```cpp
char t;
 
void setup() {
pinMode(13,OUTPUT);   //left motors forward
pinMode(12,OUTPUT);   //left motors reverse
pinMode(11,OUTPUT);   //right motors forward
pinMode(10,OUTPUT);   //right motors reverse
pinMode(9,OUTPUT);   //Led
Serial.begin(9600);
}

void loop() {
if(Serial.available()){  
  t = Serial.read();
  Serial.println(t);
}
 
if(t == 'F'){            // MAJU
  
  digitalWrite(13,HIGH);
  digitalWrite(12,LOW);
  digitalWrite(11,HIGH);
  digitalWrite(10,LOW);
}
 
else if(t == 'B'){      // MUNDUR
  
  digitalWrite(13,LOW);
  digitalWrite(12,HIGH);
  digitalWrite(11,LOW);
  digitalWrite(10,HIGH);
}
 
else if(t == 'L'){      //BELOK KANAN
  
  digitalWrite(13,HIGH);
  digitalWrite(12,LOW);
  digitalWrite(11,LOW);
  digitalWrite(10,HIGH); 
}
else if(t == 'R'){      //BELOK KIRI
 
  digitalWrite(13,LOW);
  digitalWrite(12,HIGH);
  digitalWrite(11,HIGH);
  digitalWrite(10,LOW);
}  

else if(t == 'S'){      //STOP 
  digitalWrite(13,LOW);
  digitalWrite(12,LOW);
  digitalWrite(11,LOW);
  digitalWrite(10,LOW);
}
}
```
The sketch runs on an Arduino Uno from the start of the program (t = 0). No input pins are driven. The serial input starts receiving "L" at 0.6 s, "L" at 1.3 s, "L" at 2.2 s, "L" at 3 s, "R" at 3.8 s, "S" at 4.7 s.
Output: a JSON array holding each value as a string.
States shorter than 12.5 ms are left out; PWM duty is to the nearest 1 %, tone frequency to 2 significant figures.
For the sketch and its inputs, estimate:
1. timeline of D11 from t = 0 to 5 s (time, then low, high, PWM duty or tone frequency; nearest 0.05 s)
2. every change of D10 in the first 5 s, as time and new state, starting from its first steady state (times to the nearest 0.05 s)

["0 s low; 3.8 s high; 4.7 s low", "0 s low; 0.6 s high; 3.8 s low"]
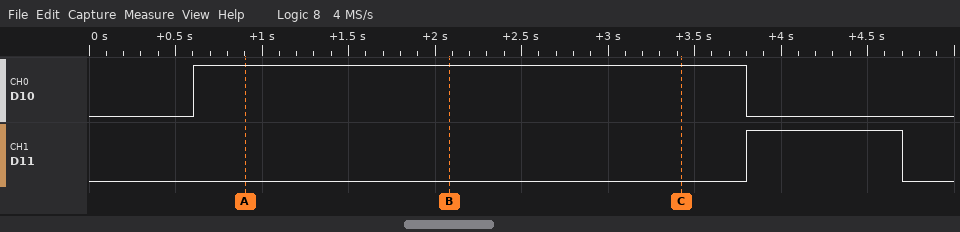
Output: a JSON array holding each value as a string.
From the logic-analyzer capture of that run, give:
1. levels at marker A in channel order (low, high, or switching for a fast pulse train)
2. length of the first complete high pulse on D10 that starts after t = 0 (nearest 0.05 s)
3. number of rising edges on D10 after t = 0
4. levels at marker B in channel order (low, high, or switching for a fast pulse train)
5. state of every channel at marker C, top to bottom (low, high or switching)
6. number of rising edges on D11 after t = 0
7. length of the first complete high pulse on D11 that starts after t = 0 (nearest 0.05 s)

["D10 high, D11 low", "3.20 s", "1", "D10 high, D11 low", "D10 high, D11 low", "1", "0.90 s"]
